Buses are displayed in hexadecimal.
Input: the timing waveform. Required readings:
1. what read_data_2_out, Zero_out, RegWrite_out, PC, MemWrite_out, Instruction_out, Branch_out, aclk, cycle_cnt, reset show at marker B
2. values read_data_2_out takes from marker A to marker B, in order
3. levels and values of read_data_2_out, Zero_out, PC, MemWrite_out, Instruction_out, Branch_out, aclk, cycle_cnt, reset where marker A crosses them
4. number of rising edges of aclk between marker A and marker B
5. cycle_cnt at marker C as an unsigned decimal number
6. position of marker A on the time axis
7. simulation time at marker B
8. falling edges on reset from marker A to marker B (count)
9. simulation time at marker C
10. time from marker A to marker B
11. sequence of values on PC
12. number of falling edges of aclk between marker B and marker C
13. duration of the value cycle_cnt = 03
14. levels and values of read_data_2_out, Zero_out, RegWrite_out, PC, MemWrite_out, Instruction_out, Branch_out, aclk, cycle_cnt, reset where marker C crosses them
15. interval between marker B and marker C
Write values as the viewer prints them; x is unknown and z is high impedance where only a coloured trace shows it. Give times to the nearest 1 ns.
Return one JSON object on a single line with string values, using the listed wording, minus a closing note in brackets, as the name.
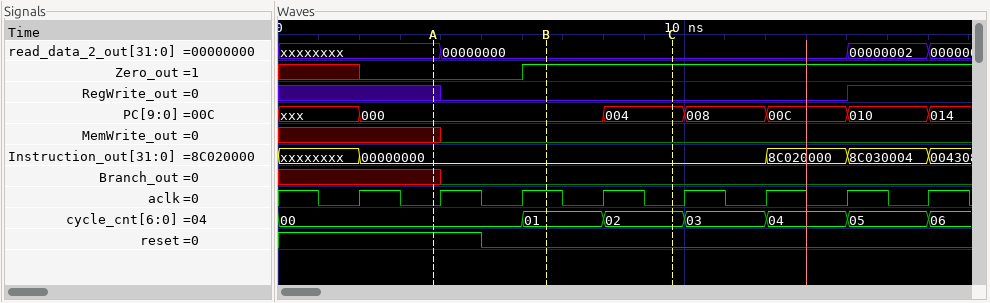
{"what read_data_2_out, Zero_out, RegWrite_out, PC, MemWrite_out, Instruction_out, Branch_out, aclk, cycle_cnt, reset show at marker B": "read_data_2_out=00000000, Zero_out=1, RegWrite_out=0, PC=000, MemWrite_out=0, Instruction_out=00000000, Branch_out=0, aclk=1, cycle_cnt=01, reset=0", "values read_data_2_out takes from marker A to marker B, in order": "xxxxxxxx, 00000000", "levels and values of read_data_2_out, Zero_out, PC, MemWrite_out, Instruction_out, Branch_out, aclk, cycle_cnt, reset where marker A crosses them": "read_data_2_out=xxxxxxxx, Zero_out=0, PC=000, MemWrite_out=x, Instruction_out=00000000, Branch_out=x, aclk=0, cycle_cnt=00, reset=1", "number of rising edges of aclk between marker A and marker B": "2", "cycle_cnt at marker C as an unsigned decimal number": "2", "position of marker A on the time axis": "4 ns", "simulation time at marker B": "7 ns", "falling edges on reset from marker A to marker B": "1", "simulation time at marker C": "10 ns", "time from marker A to marker B": "3 ns", "sequence of values on PC": "xxx, 000, 004, 008, 00C, 010, 014", "number of falling edges of aclk between marker B and marker C": "2", "duration of the value cycle_cnt = 03": "2 ns", "levels and values of read_data_2_out, Zero_out, RegWrite_out, PC, MemWrite_out, Instruction_out, Branch_out, aclk, cycle_cnt, reset where marker C crosses them": "read_data_2_out=00000000, Zero_out=1, RegWrite_out=0, PC=004, MemWrite_out=0, Instruction_out=00000000, Branch_out=0, aclk=0, cycle_cnt=02, reset=0", "interval between marker B and marker C": "3 ns"}
